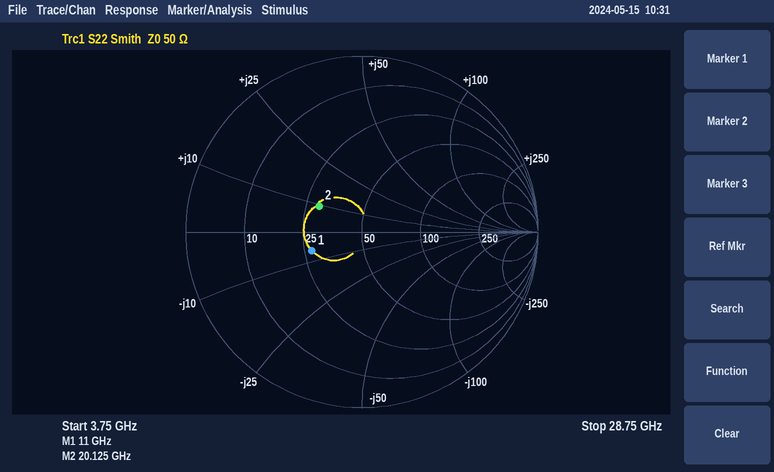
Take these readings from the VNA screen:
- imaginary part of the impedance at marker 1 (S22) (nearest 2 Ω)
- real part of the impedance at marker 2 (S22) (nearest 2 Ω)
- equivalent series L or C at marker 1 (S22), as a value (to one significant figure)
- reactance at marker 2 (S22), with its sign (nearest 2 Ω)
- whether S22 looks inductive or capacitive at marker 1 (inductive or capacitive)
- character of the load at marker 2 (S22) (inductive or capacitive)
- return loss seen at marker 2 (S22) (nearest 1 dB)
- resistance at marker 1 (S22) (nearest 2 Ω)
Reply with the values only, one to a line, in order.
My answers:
-6 Ω
30 Ω
2 pF
+10 Ω
capacitive
inductive
11 dB
28 Ω
